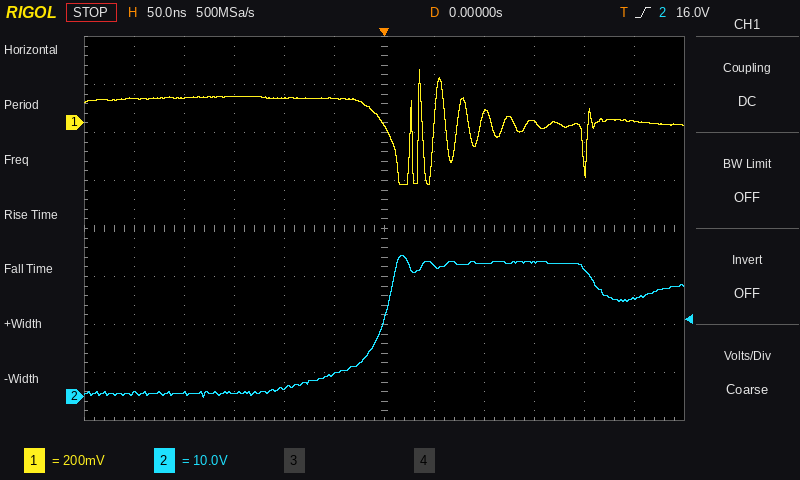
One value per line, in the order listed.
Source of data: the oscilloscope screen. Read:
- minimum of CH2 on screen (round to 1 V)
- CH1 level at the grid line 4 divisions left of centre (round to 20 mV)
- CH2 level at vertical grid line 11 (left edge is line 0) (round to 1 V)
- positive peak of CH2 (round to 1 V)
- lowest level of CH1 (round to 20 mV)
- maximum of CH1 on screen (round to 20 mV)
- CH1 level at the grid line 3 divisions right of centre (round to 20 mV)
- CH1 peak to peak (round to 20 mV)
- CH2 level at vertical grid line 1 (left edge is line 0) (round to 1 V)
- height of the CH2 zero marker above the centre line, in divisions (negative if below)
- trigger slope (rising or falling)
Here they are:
0 V
100 mV
20 V
29 V
-260 mV
220 mV
0 mV
480 mV
1 V
-3.5 div
rising
